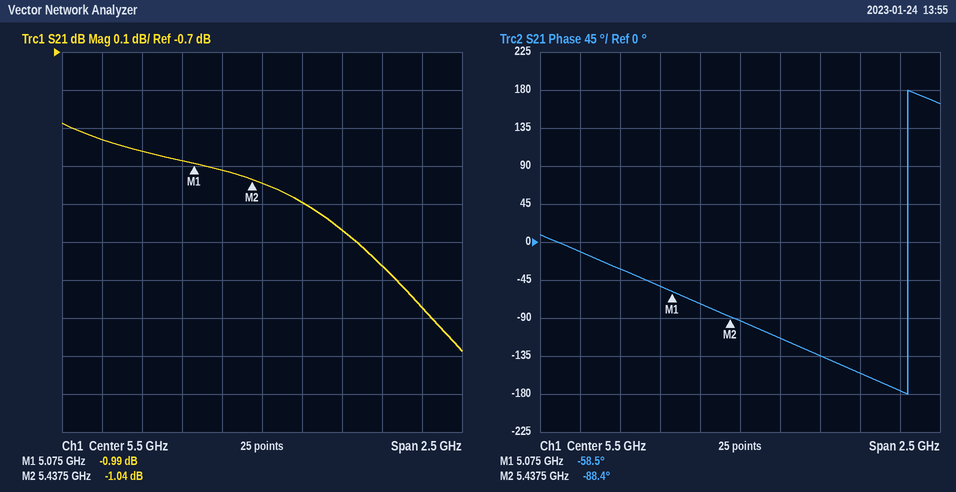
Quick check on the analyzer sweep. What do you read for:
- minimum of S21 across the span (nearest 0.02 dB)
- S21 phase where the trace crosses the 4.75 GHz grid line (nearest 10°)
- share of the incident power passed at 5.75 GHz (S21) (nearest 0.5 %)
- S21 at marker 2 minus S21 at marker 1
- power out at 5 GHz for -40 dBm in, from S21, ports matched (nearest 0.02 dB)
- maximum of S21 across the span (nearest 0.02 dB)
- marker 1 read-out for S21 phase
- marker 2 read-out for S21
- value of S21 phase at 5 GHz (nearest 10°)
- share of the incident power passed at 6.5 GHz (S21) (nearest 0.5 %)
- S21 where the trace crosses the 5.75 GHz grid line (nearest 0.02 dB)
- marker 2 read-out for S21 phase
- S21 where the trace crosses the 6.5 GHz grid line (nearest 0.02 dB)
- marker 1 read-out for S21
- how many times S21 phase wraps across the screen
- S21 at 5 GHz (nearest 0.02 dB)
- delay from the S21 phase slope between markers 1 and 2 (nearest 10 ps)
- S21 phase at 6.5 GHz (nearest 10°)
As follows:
-1.48 dB
-30°
77.5 %
-0.05 dB
-40.98 dBm
-0.88 dB
-58.5°
-1.04 dB
-50°
73.0 %
-1.10 dB
-88.4°
-1.38 dB
-0.99 dB
1
-0.98 dB
230 ps
-180°
